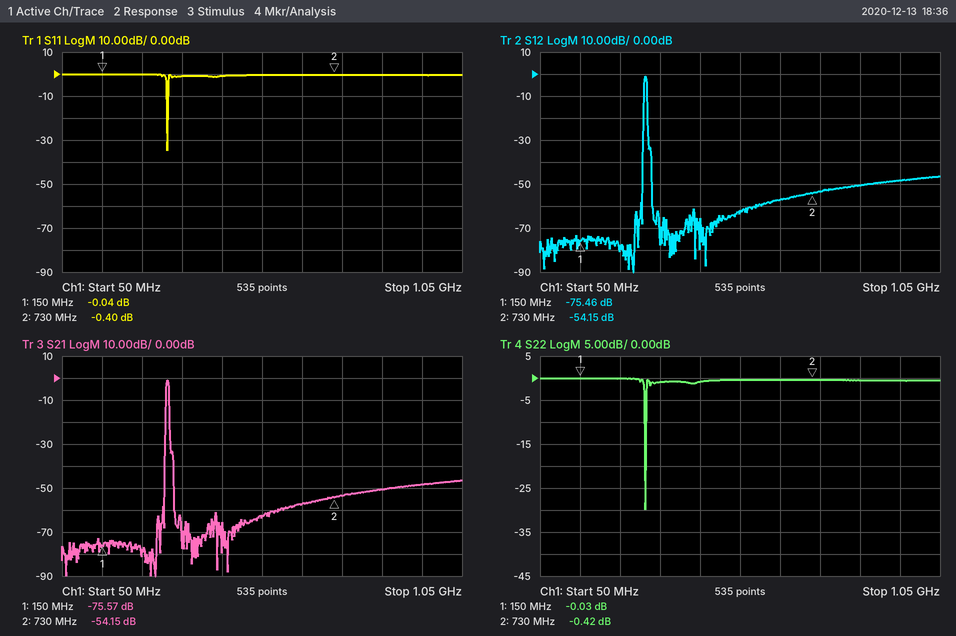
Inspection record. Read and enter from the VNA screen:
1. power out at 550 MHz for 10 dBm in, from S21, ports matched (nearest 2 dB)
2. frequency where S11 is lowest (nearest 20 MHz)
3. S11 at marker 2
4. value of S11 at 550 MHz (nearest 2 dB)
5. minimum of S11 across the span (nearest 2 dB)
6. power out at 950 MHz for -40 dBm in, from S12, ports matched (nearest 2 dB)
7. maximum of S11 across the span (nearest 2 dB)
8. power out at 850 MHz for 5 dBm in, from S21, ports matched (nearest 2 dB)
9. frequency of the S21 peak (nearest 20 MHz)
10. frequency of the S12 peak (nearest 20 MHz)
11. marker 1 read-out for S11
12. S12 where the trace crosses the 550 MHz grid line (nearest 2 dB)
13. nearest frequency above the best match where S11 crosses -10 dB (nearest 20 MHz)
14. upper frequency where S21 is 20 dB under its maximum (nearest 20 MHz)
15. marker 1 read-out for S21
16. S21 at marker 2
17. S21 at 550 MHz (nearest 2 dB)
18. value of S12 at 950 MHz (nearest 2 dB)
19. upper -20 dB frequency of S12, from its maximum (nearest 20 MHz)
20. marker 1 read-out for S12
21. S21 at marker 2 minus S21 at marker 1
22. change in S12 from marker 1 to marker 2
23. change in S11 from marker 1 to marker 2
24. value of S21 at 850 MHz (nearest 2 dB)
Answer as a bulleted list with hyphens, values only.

- -52 dBm
- 320 MHz
- -0.40 dB
- 0 dB
- -34 dB
- -88 dBm
- 0 dB
- -46 dBm
- 320 MHz
- 320 MHz
- -0.04 dB
- -62 dB
- 320 MHz
- 320 MHz
- -75.57 dB
- -54.15 dB
- -62 dB
- -48 dB
- 320 MHz
- -75.46 dB
- 21.42 dB
- 21.31 dB
- -0.36 dB
- -50 dB
